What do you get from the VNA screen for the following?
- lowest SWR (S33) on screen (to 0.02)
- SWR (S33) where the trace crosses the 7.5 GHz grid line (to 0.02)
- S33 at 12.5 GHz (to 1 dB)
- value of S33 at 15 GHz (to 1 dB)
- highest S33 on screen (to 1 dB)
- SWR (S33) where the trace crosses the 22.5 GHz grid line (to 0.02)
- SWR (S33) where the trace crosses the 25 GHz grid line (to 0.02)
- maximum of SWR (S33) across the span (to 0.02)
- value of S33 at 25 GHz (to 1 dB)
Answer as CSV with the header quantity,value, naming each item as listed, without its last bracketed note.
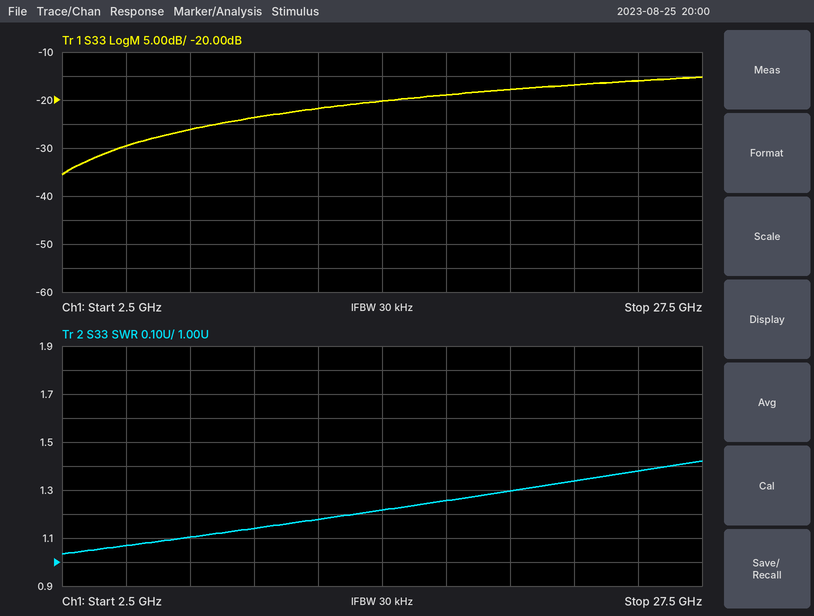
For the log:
quantity,value
lowest SWR (S33) on screen,1.04
SWR (S33) where the trace crosses the 7.5 GHz grid line,1.10
S33 at 12.5 GHz,-22 dB
value of S33 at 15 GHz,-20 dB
highest S33 on screen,-15 dB
SWR (S33) where the trace crosses the 22.5 GHz grid line,1.34
SWR (S33) where the trace crosses the 25 GHz grid line,1.38
maximum of SWR (S33) across the span,1.42
value of S33 at 25 GHz,-16 dB
